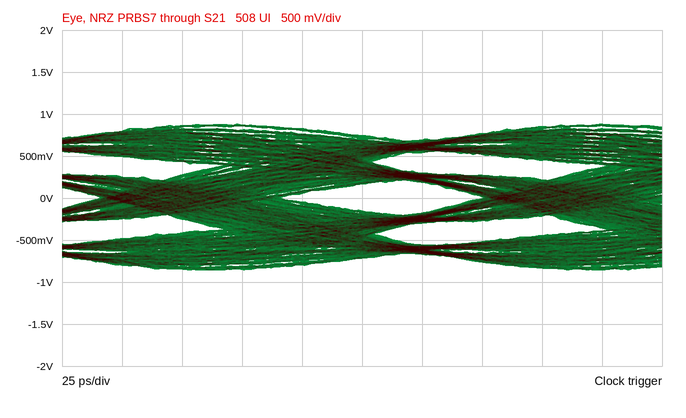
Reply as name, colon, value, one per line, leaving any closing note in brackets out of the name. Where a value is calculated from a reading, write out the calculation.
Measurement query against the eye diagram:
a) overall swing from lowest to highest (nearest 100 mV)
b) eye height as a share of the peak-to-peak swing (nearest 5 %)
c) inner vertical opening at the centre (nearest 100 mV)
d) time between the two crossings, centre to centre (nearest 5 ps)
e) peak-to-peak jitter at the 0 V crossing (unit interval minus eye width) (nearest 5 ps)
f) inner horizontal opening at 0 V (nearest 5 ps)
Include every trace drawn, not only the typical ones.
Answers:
overall swing from lowest to highest: 1.7 V
eye height as a share of the peak-to-peak swing: 300 mV / 1.7 V ≈ 17.6 %, so 20 % to the nearest 5 %
inner vertical opening at the centre: 300 mV
time between the two crossings, centre to centre: 160 ps
peak-to-peak jitter at the 0 V crossing (unit interval minus eye width): 75 ps
inner horizontal opening at 0 V: 85 ps
